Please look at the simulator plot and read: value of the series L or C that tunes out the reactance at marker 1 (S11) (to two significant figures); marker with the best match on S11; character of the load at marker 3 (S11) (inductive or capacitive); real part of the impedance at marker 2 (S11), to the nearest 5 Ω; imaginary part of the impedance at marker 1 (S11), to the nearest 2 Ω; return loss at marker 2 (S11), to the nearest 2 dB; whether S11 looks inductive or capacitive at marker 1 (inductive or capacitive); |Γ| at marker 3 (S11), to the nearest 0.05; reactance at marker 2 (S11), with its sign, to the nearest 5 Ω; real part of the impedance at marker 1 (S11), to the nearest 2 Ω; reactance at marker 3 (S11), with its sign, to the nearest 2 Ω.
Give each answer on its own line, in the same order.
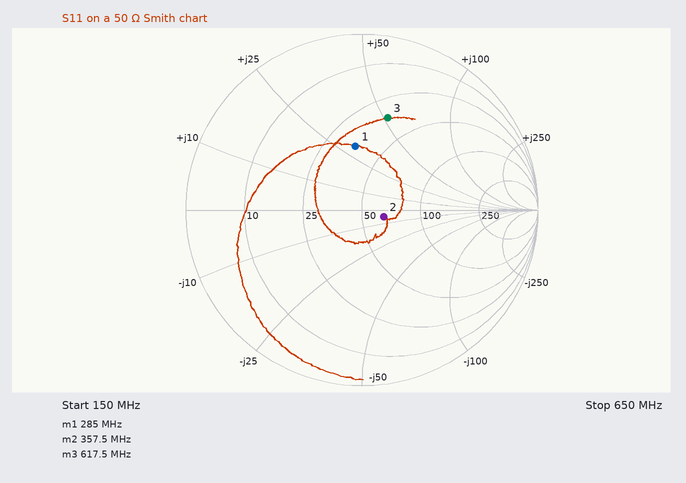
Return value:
19 pF
marker 2
inductive
65 Ω
+30 Ω
18 dB
inductive
0.55
-5 Ω
36 Ω
+52 Ω
